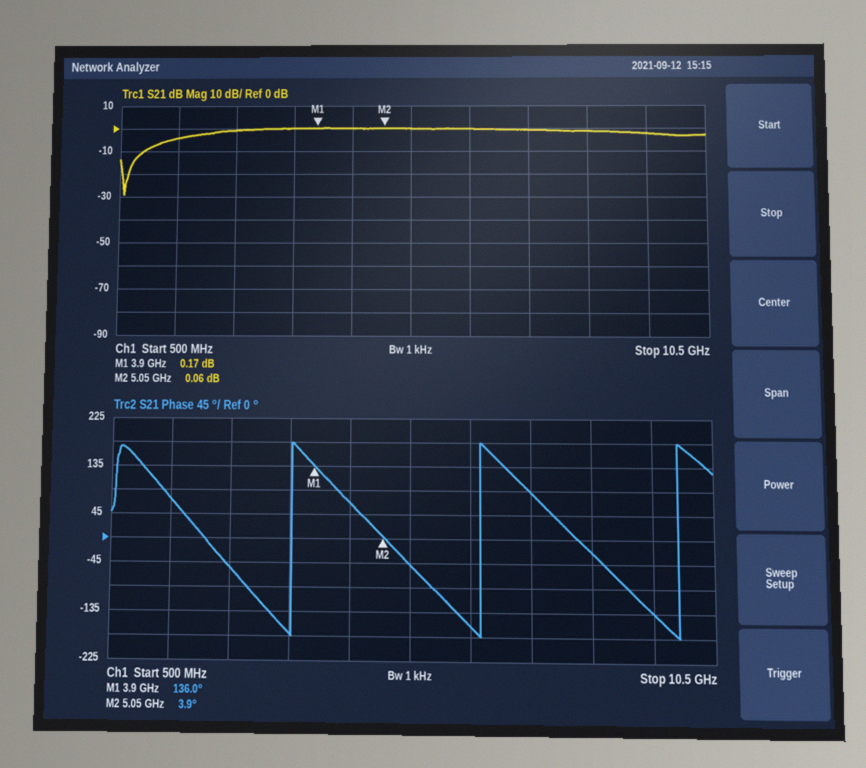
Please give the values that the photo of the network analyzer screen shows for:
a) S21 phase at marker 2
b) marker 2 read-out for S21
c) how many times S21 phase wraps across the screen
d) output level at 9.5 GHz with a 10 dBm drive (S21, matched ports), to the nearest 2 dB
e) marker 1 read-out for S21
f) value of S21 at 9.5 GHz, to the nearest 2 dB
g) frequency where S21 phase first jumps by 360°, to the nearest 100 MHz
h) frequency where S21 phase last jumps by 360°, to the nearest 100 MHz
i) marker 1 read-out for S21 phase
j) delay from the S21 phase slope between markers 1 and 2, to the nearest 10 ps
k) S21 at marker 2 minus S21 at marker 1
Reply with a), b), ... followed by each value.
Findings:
a) 3.9°
b) 0.06 dB
c) 3
d) 8 dBm
e) 0.17 dB
f) -2 dB
g) 3.5 GHz
h) 9.9 GHz
i) 136.0°
j) 320 ps
k) -0.11 dB
